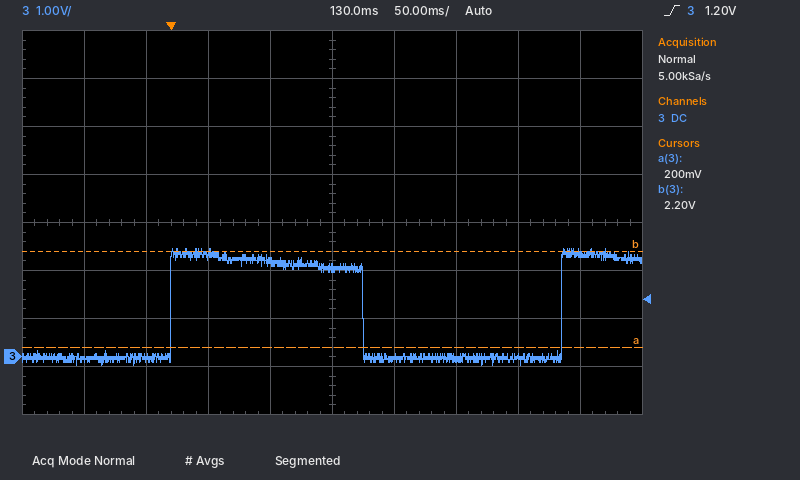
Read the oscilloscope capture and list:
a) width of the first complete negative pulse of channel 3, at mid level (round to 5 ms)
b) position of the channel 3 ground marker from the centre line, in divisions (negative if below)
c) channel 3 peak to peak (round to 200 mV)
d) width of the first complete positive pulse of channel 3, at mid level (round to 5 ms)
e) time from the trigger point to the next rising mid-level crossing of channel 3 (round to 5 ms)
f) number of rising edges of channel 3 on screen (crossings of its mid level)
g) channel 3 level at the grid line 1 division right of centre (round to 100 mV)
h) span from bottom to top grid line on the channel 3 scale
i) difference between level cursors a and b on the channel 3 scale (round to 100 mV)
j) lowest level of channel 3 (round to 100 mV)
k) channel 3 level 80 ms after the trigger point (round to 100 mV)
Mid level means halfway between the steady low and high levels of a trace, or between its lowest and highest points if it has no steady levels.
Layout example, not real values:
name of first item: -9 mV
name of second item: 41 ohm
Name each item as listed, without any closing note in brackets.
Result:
width of the first complete negative pulse of channel 3, at mid level: 160 ms
position of the channel 3 ground marker from the centre line, in divisions: -2.8 div
channel 3 peak to peak: 2.4 V
width of the first complete positive pulse of channel 3, at mid level: 155 ms
time from the trigger point to the next rising mid-level crossing of channel 3: 315 ms
number of rising edges of channel 3 on screen: 2
channel 3 level at the grid line 1 division right of centre: 0.0 V
span from bottom to top grid line on the channel 3 scale: 8 V
difference between level cursors a and b on the channel 3 scale: 2.0 V
lowest level of channel 3: -200 mV
channel 3 level 80 ms after the trigger point: 2.0 V
